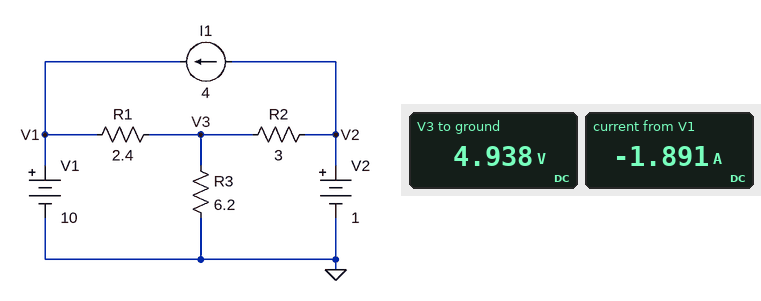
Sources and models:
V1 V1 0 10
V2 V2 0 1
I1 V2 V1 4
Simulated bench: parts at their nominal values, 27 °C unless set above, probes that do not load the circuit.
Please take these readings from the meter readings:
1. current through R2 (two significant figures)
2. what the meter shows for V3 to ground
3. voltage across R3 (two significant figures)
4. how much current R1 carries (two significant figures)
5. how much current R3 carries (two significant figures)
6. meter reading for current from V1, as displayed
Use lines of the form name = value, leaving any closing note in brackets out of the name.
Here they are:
current through R2 = 1.3 A
what the meter shows for V3 to ground = 4.938 V
voltage across R3 = 4.9 V
how much current R1 carries = 2.1 A
how much current R3 carries = 800 mA
meter reading for current from V1, as displayed = -1.891 A
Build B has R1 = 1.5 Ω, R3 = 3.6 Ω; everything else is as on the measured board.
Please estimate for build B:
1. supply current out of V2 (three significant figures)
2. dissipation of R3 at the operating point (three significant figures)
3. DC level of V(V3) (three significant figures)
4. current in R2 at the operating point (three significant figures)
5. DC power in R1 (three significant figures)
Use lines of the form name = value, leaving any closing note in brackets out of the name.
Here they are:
supply current out of V2 = 2.51 A
dissipation of R3 at the operating point = 8.34 W
DC level of V(V3) = 5.48 V
current in R2 at the operating point = 1.49 A
DC power in R1 = 13.6 W
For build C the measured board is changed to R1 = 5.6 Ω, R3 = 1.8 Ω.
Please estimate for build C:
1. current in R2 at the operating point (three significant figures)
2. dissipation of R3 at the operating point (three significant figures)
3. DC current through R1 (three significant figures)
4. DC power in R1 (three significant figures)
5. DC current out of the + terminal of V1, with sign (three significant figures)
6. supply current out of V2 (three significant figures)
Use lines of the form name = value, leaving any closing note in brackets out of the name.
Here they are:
current in R2 at the operating point = 328 mA
dissipation of R3 at the operating point = 2.19 W
DC current through R1 = 1.43 A
DC power in R1 = 11.5 W
DC current out of the + terminal of V1, with sign = -2.57 A
supply current out of V2 = 3.67 A
